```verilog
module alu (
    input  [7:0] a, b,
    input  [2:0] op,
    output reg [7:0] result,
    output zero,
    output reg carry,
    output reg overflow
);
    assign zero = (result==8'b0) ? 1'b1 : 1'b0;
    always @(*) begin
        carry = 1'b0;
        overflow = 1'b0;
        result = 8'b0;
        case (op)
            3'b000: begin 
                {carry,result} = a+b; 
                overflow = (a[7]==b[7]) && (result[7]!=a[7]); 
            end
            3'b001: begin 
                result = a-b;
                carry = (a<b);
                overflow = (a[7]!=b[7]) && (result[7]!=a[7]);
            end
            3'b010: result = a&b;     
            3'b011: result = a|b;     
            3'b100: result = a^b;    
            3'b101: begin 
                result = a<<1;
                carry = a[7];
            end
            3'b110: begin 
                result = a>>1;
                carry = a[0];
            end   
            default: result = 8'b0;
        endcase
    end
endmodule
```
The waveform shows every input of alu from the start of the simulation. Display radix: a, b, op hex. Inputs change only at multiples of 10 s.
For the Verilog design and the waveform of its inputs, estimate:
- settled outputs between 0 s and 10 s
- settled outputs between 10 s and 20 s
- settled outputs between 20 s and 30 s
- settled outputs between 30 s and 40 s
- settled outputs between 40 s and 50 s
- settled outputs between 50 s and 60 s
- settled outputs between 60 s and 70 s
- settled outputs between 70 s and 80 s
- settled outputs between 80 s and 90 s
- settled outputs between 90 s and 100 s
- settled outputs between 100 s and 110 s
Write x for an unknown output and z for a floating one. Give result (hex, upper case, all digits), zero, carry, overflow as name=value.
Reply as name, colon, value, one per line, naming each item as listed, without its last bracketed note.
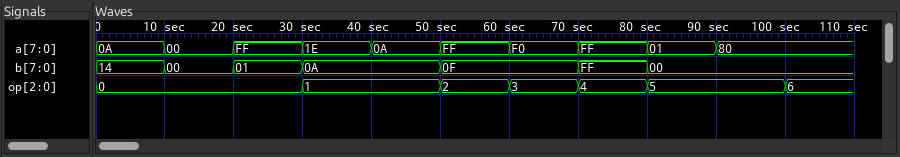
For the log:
settled outputs between 0 s and 10 s: result=1E, zero=0, carry=0, overflow=0
settled outputs between 10 s and 20 s: result=00, zero=1, carry=0, overflow=0
settled outputs between 20 s and 30 s: result=00, zero=1, carry=1, overflow=0
settled outputs between 30 s and 40 s: result=14, zero=0, carry=0, overflow=0
settled outputs between 40 s and 50 s: result=00, zero=1, carry=0, overflow=0
settled outputs between 50 s and 60 s: result=0F, zero=0, carry=0, overflow=0
settled outputs between 60 s and 70 s: result=FF, zero=0, carry=0, overflow=0
settled outputs between 70 s and 80 s: result=00, zero=1, carry=0, overflow=0
settled outputs between 80 s and 90 s: result=02, zero=0, carry=0, overflow=0
settled outputs between 90 s and 100 s: result=00, zero=1, carry=1, overflow=0
settled outputs between 100 s and 110 s: result=40, zero=0, carry=0, overflow=0
